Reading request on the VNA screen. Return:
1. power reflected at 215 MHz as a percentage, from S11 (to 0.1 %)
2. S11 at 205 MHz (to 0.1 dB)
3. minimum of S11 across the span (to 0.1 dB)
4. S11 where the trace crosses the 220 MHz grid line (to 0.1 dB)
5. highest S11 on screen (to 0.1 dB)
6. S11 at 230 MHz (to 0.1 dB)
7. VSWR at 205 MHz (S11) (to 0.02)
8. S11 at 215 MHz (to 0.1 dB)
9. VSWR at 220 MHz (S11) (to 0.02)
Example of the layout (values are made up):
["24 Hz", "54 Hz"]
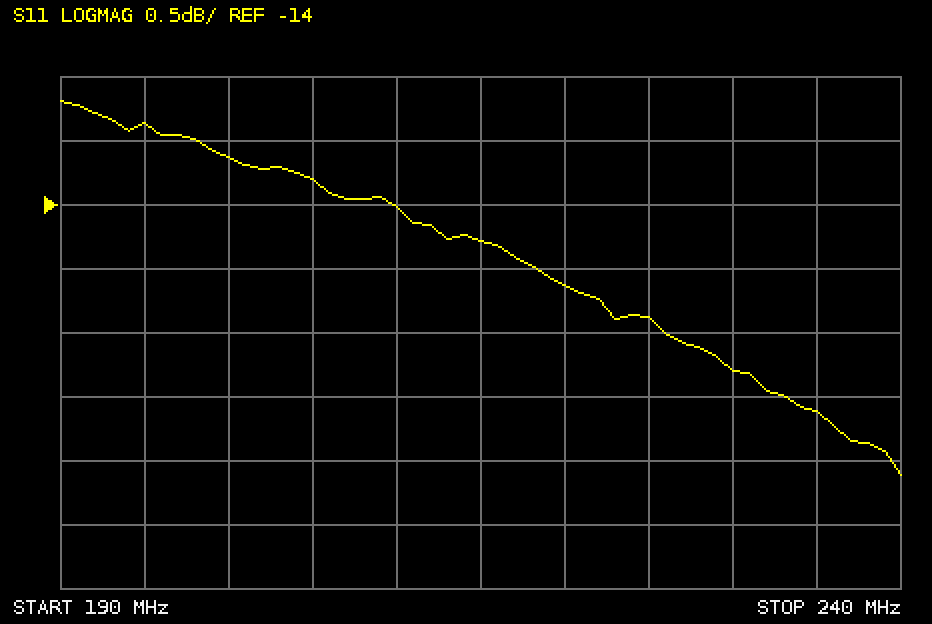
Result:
["3.7 %", "-13.8 dB", "-16.1 dB", "-14.6 dB", "-13.2 dB", "-15.3 dB", "1.52", "-14.3 dB", "1.46"]
